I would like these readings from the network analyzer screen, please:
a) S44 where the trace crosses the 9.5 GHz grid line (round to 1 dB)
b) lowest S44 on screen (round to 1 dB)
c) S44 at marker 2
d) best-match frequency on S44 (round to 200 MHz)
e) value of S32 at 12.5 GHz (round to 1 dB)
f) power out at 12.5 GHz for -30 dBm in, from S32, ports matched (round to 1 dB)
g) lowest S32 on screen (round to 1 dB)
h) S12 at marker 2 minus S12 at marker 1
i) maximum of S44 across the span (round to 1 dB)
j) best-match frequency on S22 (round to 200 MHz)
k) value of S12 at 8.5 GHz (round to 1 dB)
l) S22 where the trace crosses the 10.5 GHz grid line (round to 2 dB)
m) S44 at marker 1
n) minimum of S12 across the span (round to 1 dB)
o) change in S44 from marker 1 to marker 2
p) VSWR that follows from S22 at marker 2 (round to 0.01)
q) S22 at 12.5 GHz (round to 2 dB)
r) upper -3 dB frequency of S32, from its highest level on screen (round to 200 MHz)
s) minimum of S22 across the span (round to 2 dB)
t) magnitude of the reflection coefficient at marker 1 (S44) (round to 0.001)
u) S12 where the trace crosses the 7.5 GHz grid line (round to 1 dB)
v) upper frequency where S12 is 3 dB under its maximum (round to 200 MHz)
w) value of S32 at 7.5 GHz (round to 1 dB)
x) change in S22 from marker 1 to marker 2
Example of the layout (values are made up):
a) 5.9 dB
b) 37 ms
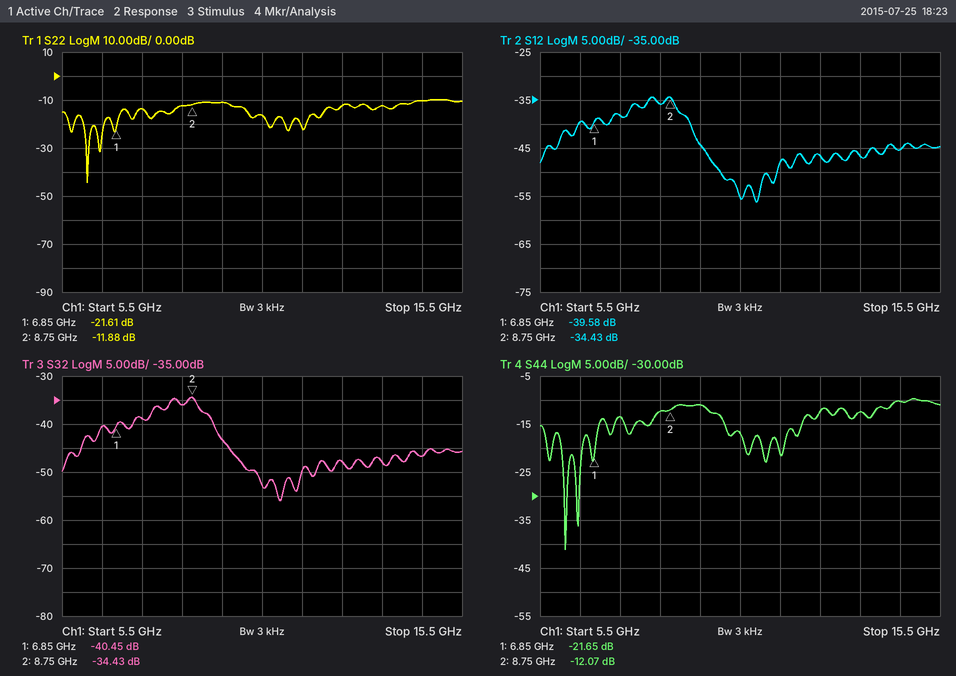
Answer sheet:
a) -11 dB
b) -41 dB
c) -12.07 dB
d) 6.2 GHz
e) -48 dB
f) -78 dBm
g) -56 dB
h) 5.15 dB
i) -10 dB
j) 6.2 GHz
k) -36 dB
l) -16 dB
m) -21.65 dB
n) -56 dB
o) 9.58 dB
p) 1.68
q) -12 dB
r) 9.0 GHz
s) -44 dB
t) 0.083
u) -38 dB
v) 9.0 GHz
w) -39 dB
x) 9.73 dB
